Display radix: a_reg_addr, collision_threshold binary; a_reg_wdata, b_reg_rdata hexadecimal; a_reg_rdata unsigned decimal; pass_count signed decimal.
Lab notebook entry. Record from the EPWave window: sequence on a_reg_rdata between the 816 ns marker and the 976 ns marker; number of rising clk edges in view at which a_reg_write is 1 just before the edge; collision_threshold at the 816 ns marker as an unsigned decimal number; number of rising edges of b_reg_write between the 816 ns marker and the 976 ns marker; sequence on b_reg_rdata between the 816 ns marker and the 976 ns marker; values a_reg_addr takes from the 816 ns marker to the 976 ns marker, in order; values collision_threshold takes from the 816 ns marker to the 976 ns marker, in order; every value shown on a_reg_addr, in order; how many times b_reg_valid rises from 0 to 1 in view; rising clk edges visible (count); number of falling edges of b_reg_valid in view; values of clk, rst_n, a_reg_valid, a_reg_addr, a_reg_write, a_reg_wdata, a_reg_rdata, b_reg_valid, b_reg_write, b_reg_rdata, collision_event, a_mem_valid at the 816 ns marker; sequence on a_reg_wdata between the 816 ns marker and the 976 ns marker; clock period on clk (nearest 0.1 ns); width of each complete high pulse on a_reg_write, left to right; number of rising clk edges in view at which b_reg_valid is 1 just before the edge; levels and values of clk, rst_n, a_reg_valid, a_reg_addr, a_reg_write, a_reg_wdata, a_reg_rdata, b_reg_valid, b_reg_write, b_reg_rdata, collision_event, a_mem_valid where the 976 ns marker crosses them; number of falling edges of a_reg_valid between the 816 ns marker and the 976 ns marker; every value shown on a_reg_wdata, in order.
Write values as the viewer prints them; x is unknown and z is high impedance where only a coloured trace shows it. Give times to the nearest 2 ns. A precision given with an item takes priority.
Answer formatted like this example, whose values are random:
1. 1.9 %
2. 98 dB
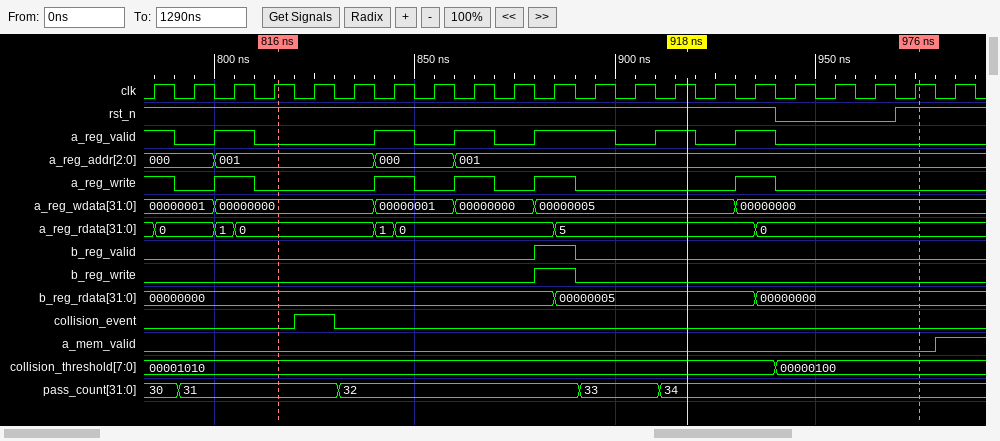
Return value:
1. 0, 1, 0, 5, 0
2. 6
3. 10
4. 1
5. 00000000, 00000005, 00000000
6. 001, 000, 001
7. 00001010, 00000100
8. 000, 001, 000, 001
9. 1
10. 21
11. 1
12. clk=1, rst_n=1, a_reg_valid=0, a_reg_addr=001, a_reg_write=0, a_reg_wdata=00000000, a_reg_rdata=0, b_reg_valid=0, b_reg_write=0, b_reg_rdata=00000000, collision_event=0, a_mem_valid=0
13. 00000000, 00000001, 00000000, 00000005, 00000000
14. 10 ns
15. 10 ns, 10 ns, 10 ns, 10 ns, 10 ns
16. 1
17. clk=1, rst_n=1, a_reg_valid=0, a_reg_addr=001, a_reg_write=0, a_reg_wdata=00000000, a_reg_rdata=0, b_reg_valid=0, b_reg_write=0, b_reg_rdata=00000000, collision_event=0, a_mem_valid=0
18. 5
19. 00000001, 00000000, 00000001, 00000000, 00000005, 00000000
